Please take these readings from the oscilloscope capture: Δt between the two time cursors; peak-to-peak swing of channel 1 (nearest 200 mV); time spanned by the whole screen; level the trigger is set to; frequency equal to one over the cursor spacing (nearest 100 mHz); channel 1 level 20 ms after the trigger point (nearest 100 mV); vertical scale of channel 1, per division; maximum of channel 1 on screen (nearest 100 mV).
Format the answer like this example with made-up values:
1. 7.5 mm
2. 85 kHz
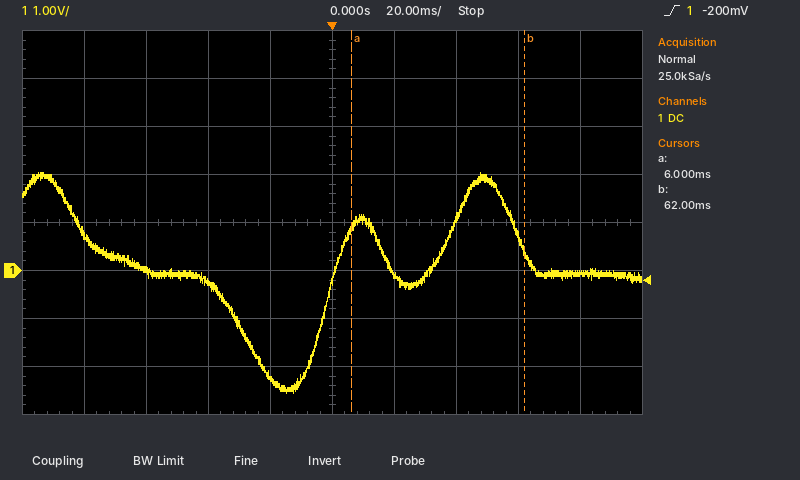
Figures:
1. 56 ms
2. 4.6 V
3. 200 ms
4. -200 mV
5. 17.9 Hz
6. -100 mV
7. 1 V
8. 2.0 V
